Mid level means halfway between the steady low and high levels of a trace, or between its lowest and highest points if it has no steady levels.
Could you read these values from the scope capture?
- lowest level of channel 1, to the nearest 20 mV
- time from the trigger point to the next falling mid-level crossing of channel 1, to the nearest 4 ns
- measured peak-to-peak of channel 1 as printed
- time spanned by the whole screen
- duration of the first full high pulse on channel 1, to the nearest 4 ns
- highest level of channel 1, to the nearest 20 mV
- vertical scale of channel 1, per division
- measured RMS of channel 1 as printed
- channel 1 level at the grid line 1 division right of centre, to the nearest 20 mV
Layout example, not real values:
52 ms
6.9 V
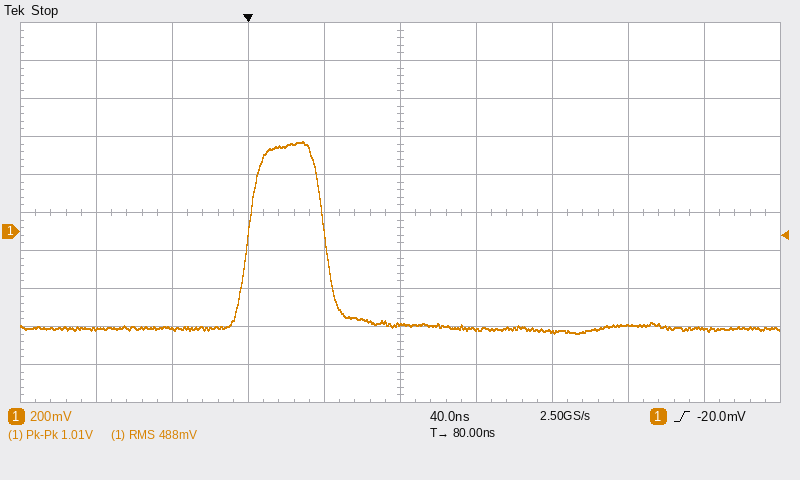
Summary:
-540 mV
40 ns
1.01 V
400 ns
40 ns
480 mV
200 mV
488 mV
-520 mV
